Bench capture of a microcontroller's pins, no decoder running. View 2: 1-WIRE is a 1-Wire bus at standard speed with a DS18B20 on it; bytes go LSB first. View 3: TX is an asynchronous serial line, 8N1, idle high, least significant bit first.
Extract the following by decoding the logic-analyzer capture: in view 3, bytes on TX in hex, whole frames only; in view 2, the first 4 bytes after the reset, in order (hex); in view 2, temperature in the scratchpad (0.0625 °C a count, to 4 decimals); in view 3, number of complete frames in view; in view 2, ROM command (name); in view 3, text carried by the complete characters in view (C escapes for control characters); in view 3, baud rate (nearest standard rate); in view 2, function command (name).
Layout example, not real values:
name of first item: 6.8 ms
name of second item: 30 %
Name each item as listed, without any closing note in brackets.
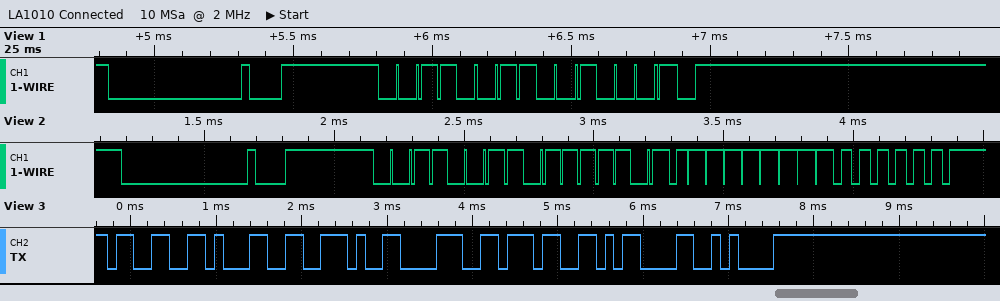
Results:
in view 3, bytes on TX in hex, whole frames only: 0x33 0x31 0x2E 0x38 0x37 0x0D 0x0A
in view 2, the first 4 bytes after the reset, in order: CC BE FE 01
in view 2, temperature in the scratchpad: 31.8750 °C
in view 3, number of complete frames in view: 7
in view 2, ROM command: Skip ROM
in view 3, text carried by the complete characters in view: "31.87\r\n"
in view 3, baud rate: 9600 baud
in view 2, function command: Read Scratchpad
